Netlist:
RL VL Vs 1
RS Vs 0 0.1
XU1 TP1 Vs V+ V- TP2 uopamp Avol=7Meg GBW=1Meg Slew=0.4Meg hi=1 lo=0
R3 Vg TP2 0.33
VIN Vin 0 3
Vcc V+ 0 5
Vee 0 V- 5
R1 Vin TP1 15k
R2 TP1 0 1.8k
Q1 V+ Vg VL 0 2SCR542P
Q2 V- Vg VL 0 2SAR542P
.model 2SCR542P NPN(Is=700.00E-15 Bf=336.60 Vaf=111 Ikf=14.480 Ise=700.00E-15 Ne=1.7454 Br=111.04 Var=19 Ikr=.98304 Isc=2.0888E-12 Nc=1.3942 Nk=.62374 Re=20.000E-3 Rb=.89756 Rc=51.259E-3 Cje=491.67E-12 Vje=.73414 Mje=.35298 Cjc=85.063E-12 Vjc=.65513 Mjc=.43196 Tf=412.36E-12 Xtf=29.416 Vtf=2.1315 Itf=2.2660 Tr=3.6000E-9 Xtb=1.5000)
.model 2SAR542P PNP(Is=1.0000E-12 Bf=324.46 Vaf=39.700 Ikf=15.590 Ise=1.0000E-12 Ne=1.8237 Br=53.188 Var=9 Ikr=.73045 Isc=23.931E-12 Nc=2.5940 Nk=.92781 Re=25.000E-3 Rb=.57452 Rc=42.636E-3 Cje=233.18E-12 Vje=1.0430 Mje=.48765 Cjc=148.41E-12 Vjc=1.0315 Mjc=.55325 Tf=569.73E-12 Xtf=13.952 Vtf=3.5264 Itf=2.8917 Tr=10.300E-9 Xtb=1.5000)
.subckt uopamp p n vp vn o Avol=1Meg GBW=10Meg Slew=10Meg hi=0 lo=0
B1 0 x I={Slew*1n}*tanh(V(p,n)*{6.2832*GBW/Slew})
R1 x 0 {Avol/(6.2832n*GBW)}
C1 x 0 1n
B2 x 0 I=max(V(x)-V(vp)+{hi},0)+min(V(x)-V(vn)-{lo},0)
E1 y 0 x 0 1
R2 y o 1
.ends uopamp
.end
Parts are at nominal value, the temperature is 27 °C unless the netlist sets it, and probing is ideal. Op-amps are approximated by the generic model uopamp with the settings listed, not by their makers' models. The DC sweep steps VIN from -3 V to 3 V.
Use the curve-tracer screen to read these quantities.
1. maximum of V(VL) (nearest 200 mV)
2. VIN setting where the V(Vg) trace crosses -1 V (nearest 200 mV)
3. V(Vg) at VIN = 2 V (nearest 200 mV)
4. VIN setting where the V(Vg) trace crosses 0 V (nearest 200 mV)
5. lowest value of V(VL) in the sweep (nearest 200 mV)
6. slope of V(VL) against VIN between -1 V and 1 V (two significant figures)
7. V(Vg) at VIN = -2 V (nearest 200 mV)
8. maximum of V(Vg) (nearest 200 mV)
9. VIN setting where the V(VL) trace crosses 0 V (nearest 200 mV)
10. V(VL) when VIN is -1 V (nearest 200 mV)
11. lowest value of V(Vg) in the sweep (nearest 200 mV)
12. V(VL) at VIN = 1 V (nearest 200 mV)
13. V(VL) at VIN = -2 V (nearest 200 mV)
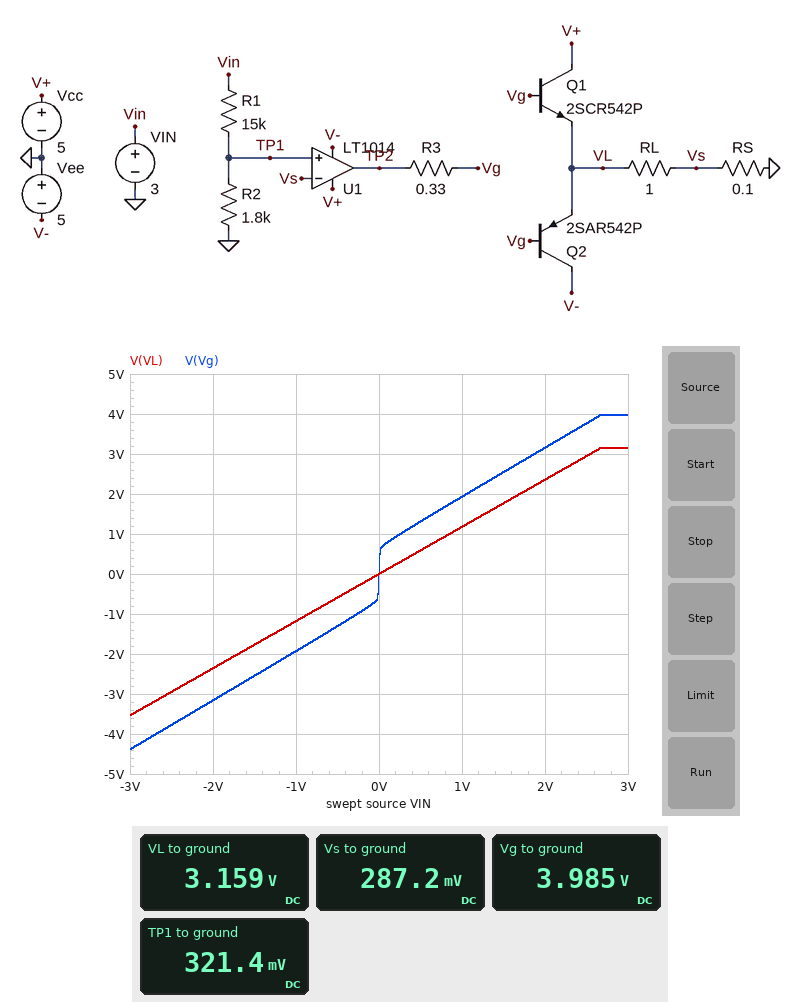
3.2 V
-200 mV
3.2 V
0 V
-3.6 V
1.2 V/V
-3.2 V
4.0 V
0 V
-1.2 V
-4.4 V
1.2 V
-2.4 V
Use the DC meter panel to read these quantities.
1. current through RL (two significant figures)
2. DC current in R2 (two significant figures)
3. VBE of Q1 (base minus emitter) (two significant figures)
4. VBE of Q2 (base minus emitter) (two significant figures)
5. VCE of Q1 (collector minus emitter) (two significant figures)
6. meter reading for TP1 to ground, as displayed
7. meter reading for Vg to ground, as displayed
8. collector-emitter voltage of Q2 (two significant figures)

2.9 A
180 µA
830 mV
830 mV
1.8 V
321.4 mV
3.985 V
-8.2 V
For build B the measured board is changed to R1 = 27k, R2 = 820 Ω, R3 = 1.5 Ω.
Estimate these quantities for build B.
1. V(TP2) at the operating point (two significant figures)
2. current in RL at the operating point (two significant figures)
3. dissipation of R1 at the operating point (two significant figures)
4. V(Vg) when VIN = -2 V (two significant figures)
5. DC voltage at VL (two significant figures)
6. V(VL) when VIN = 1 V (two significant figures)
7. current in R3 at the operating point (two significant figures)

1.7 V
880 mA
310 µW
-1.4 V
970 mV
320 mV
2.9 mA
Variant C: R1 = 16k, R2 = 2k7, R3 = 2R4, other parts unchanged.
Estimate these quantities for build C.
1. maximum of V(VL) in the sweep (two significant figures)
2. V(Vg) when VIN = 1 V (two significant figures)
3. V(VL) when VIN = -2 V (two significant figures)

3.1 V
2.4 V
-3.2 V
